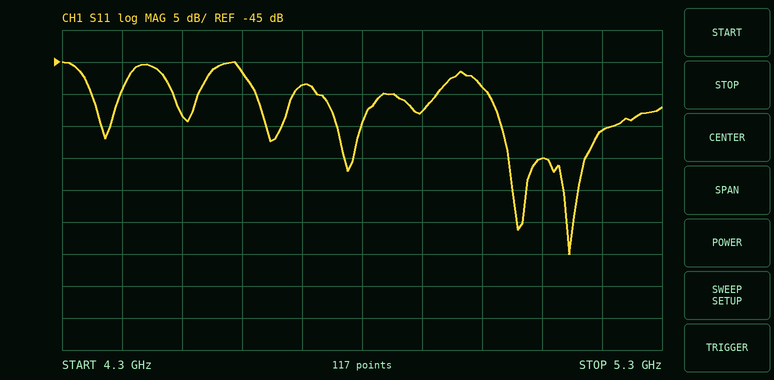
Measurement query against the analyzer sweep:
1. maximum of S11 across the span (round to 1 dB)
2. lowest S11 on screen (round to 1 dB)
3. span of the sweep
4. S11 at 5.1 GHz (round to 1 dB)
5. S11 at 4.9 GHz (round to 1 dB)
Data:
-45 dB
-75 dB
1 GHz
-60 dB
-53 dB
